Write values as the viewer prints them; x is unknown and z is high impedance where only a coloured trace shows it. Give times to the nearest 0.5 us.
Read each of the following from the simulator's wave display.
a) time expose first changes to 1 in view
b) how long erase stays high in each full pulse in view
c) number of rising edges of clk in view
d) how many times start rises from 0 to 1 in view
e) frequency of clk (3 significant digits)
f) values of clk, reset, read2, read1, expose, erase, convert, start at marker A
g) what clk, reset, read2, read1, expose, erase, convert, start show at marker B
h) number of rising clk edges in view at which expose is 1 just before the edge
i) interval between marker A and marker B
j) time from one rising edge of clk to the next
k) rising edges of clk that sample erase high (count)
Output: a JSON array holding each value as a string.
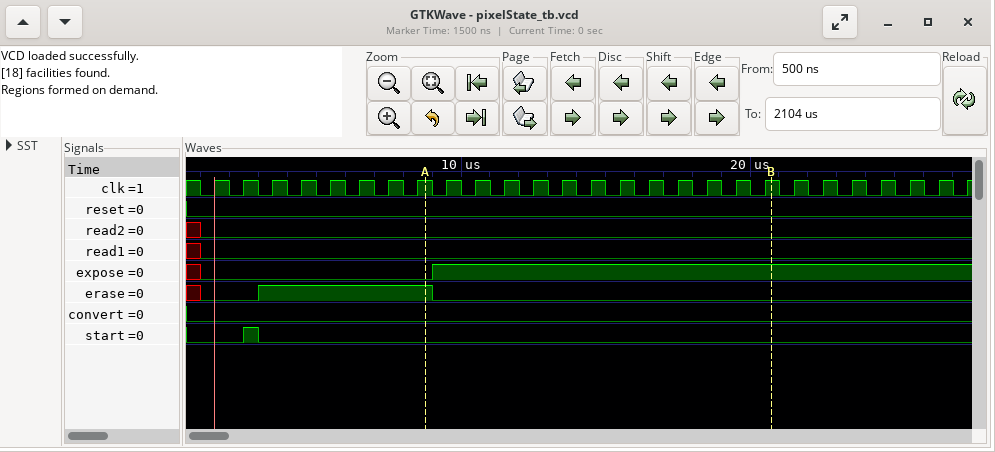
["9 us", "6 us", "27", "1", "1.00 MHz", "clk=1, reset=0, read2=0, read1=0, expose=0, erase=1, convert=0, start=0", "clk=1, reset=0, read2=0, read1=0, expose=1, erase=0, convert=0, start=0", "19", "12 us", "1 us", "6"]
